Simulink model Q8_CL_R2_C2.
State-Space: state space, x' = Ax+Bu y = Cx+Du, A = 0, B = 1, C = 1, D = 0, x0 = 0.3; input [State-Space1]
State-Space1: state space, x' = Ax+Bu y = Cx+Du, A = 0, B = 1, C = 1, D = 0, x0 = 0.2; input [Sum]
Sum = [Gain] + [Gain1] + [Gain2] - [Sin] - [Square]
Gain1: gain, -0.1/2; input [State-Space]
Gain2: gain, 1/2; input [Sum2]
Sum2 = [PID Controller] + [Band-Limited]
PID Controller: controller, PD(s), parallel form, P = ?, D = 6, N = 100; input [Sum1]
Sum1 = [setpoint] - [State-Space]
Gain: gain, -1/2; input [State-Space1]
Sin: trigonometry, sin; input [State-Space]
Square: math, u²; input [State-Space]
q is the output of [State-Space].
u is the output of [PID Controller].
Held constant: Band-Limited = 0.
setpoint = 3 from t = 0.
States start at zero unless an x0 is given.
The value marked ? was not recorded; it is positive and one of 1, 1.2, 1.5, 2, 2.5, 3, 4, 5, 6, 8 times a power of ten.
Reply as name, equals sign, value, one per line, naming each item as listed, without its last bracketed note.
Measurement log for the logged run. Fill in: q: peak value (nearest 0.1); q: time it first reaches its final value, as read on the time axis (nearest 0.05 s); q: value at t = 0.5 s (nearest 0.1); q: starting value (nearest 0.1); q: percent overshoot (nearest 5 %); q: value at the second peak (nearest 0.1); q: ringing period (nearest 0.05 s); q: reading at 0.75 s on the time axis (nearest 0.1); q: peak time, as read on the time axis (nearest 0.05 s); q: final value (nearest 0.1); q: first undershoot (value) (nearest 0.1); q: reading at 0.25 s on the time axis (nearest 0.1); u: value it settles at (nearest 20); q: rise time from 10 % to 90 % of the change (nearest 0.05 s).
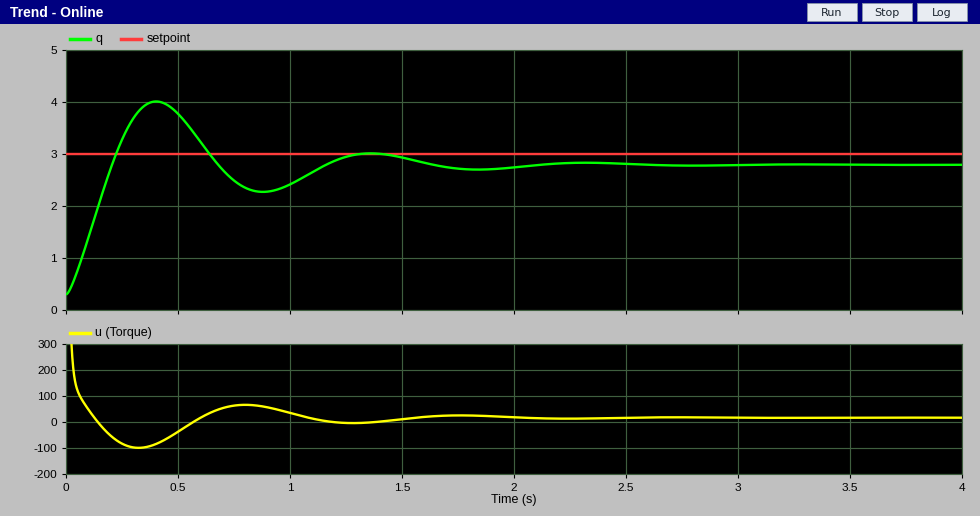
q: peak value = 4.0
q: time it first reaches its final value, as read on the time axis = 0.20 s
q: value at t = 0.5 s = 3.8
q: starting value = 0.3
q: percent overshoot = 50 %
q: value at the second peak = 3.0
q: ringing period = 0.95 s
q: reading at 0.75 s on the time axis = 2.5
q: peak time, as read on the time axis = 0.40 s
q: final value = 2.8
q: first undershoot (value) = 2.3
q: reading at 0.25 s on the time axis = 3.3
u: value it settles at = 20
q: rise time from 10 % to 90 % of the change = 0.15 s
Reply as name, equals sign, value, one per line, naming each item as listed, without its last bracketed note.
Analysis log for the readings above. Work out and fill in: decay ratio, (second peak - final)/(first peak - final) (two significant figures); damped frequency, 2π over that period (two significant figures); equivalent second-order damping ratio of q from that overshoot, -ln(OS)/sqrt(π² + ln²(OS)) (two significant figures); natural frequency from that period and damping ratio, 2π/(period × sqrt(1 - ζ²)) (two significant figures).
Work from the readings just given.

decay ratio, (second peak - final)/(first peak - final) = 0.17
damped frequency, 2π over that period = 6.6 rad/s
equivalent second-order damping ratio of q from that overshoot, -ln(OS)/sqrt(π² + ln²(OS)) = 0.22
natural frequency from that period and damping ratio, 2π/(period × sqrt(1 - ζ²)) = 6.8 rad/s
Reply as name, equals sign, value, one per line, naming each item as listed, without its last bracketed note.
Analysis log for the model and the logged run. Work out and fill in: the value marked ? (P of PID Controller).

the value marked ? = 80
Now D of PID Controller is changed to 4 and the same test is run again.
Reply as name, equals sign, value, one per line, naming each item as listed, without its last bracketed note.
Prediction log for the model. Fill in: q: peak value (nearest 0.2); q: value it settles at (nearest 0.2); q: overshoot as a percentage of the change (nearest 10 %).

q: peak value = 4.2
q: value it settles at = 2.8
q: overshoot as a percentage of the change = 60 %
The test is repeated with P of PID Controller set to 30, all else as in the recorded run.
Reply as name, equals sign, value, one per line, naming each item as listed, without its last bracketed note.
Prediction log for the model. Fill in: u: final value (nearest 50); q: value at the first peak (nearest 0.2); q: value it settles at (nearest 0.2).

u: final value = 0
q: value at the first peak = 3.4
q: value it settles at = 2.6
